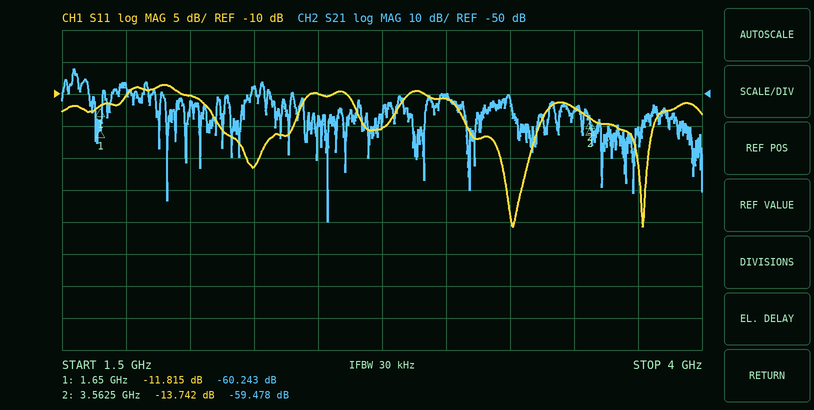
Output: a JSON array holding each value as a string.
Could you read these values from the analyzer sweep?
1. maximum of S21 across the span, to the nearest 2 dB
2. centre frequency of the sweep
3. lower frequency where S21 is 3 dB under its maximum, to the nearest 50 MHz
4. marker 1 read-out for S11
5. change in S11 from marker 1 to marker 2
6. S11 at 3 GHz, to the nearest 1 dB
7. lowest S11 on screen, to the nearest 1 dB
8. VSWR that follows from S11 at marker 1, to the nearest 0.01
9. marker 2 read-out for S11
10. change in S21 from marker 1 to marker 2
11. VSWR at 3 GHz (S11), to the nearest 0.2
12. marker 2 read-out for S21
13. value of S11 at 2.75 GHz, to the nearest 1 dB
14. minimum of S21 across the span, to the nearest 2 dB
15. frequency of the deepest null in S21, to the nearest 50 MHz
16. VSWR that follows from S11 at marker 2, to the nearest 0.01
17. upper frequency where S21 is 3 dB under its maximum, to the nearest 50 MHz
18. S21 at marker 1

["-42 dB", "2.75 GHz", "1.55 GHz", "-11.815 dB", "-1.927 dB", "-11 dB", "-31 dB", "1.69", "-13.742 dB", "0.765 dB", "1.8", "-59.478 dB", "-15 dB", "-90 dB", "2.55 GHz", "1.52", "1.55 GHz", "-60.243 dB"]
